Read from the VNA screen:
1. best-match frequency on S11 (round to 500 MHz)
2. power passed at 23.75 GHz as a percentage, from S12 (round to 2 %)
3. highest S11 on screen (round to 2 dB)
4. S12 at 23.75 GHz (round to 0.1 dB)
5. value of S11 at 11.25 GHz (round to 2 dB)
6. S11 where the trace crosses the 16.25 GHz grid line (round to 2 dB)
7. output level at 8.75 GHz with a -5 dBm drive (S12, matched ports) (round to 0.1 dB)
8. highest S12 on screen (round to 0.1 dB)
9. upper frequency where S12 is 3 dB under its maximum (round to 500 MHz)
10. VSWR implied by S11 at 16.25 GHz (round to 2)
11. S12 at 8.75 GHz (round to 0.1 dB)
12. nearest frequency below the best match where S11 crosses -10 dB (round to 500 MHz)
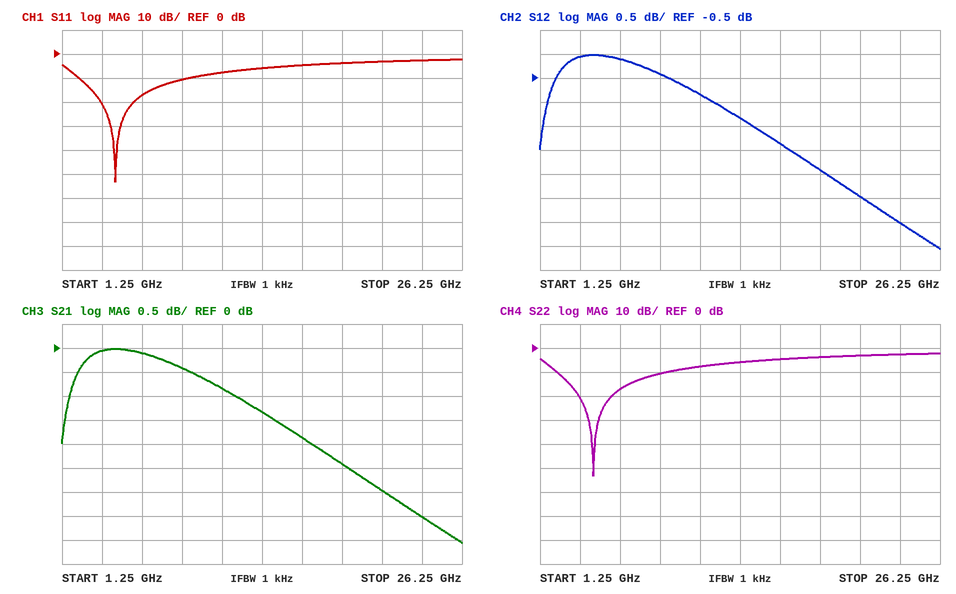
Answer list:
4.5 GHz
44 %
-2 dB
-3.5 dB
-8 dB
-4 dB
-5.4 dBm
0.0 dB
21.5 GHz
4
-0.4 dB
2.5 GHz
